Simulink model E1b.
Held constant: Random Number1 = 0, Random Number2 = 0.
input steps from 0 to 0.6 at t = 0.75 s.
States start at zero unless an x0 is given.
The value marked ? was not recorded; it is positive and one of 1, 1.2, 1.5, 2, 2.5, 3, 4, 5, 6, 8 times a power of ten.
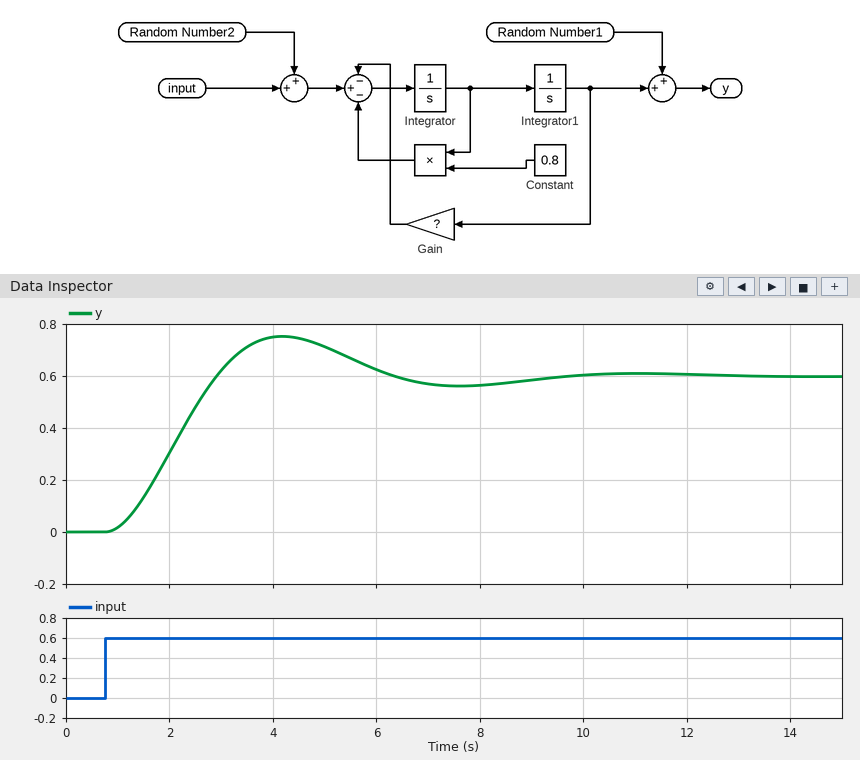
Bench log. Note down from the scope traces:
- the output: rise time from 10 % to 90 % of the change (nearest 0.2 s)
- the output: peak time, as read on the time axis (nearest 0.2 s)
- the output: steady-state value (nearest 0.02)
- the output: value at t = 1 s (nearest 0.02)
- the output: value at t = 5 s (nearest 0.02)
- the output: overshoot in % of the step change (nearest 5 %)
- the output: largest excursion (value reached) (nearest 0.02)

1.4 s
4.2 s
0.60
0.02
0.72
25 %
0.76
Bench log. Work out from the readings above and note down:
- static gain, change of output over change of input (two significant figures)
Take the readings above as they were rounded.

1.0
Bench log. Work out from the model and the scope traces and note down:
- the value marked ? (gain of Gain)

1
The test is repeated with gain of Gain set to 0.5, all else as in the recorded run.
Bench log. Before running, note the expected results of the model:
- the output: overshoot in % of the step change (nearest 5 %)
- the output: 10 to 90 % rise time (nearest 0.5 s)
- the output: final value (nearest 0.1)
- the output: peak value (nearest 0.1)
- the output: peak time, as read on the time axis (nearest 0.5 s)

10 %
2.5 s
1.2
1.3
6.0 s
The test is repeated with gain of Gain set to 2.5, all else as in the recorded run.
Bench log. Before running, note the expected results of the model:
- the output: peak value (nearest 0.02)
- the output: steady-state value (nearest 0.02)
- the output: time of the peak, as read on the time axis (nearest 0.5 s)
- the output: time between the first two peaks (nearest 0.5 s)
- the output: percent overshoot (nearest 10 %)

0.34
0.24
3.0 s
4.0 s
40 %
